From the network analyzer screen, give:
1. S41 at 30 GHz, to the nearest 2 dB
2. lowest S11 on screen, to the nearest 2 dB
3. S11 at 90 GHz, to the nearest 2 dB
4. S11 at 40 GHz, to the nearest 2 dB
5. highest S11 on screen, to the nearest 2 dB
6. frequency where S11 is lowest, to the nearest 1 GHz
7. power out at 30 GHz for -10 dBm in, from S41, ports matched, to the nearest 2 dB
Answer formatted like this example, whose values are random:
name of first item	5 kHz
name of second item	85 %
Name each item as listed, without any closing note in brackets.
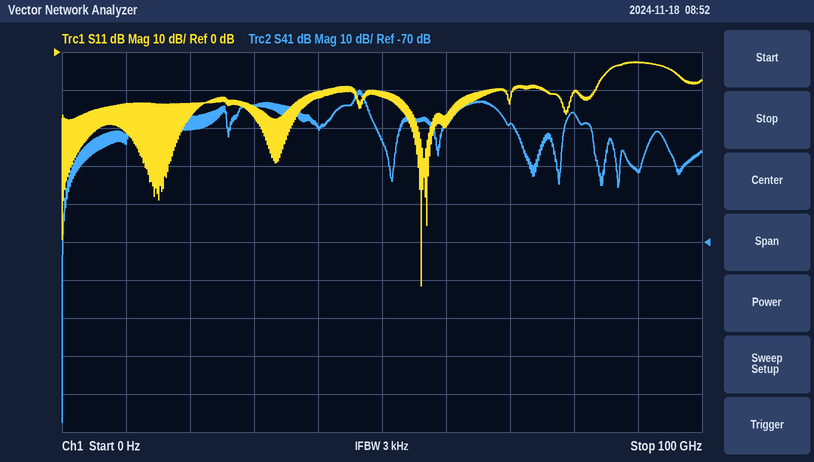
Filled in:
S41 at 30 GHz, to the nearest 2 dB	-34 dB
lowest S11 on screen, to the nearest 2 dB	-62 dB
S11 at 90 GHz, to the nearest 2 dB	-2 dB
S11 at 40 GHz, to the nearest 2 dB	-12 dB
highest S11 on screen, to the nearest 2 dB	-2 dB
frequency where S11 is lowest, to the nearest 1 GHz	56 GHz
power out at 30 GHz for -10 dBm in, from S41, ports matched, to the nearest 2 dB	-44 dBm
